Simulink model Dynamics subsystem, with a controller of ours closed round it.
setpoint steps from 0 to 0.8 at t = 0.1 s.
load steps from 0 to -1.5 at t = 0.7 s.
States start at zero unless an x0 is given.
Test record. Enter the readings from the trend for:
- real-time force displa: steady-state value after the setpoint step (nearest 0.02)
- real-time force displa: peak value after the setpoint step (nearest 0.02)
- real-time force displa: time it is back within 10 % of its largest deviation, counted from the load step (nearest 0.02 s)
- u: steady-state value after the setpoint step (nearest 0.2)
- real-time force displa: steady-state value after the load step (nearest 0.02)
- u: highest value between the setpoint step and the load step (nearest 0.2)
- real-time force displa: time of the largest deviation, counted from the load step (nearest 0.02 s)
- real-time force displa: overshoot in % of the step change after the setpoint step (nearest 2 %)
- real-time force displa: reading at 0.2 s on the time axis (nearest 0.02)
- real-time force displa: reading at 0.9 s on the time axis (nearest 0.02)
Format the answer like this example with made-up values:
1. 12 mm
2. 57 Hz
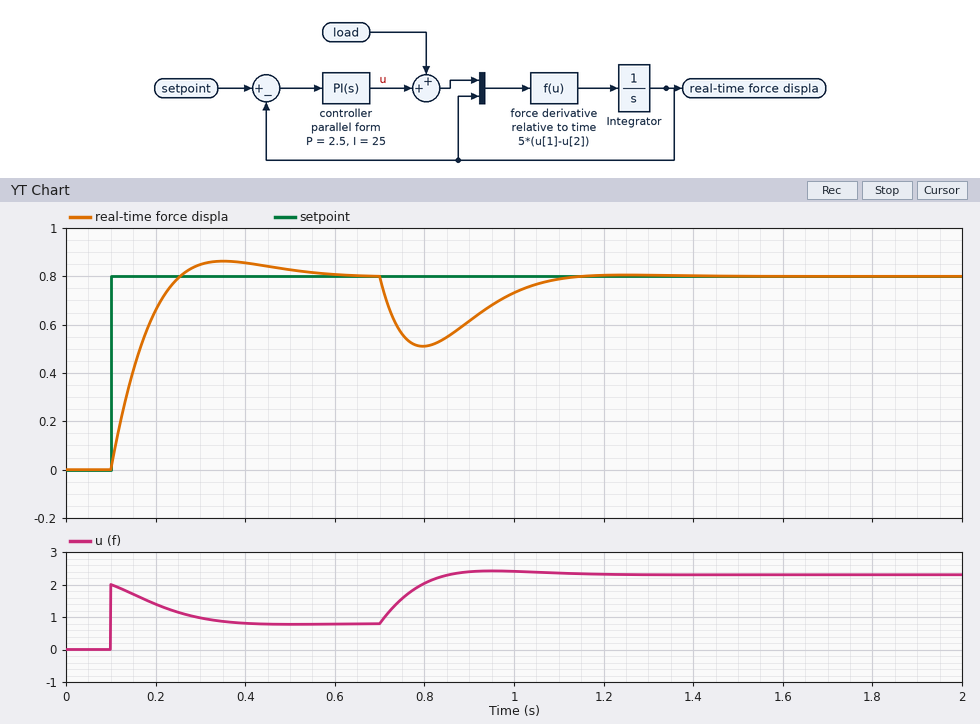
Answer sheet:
1. 0.80
2. 0.86
3. 0.36 s
4. 0.8
5. 0.80
6. 2.0
7. 0.10 s
8. 8 %
9. 0.66
10. 0.62
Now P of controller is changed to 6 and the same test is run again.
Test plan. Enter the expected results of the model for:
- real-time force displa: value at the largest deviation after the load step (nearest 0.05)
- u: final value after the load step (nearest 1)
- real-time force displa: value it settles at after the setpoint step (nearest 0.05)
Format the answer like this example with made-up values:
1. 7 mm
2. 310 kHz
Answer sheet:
1. 0.60
2. 2
3. 0.80
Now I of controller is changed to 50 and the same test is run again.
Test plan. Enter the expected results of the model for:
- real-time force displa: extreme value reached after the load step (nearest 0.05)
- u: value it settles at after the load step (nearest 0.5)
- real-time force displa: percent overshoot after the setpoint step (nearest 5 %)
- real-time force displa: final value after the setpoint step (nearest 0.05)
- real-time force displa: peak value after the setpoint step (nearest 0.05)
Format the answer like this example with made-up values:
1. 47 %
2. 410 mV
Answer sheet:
1. 0.55
2. 2.5
3. 20 %
4. 0.80
5. 0.95
